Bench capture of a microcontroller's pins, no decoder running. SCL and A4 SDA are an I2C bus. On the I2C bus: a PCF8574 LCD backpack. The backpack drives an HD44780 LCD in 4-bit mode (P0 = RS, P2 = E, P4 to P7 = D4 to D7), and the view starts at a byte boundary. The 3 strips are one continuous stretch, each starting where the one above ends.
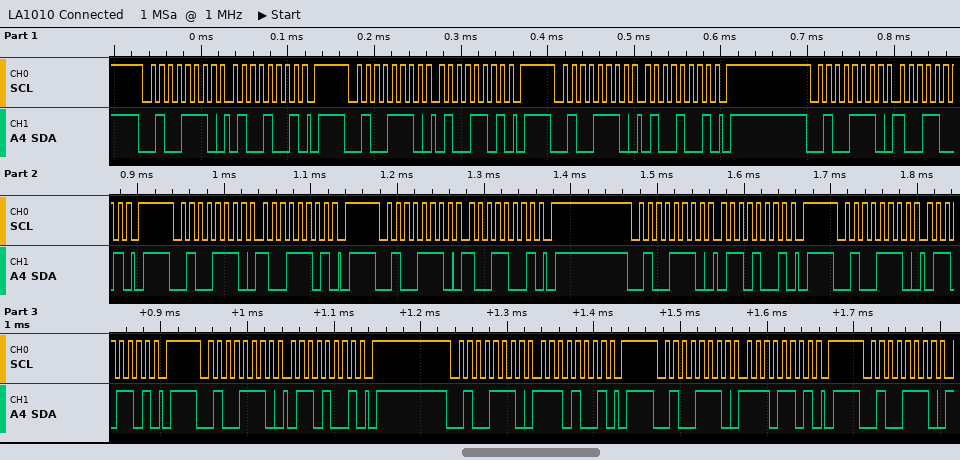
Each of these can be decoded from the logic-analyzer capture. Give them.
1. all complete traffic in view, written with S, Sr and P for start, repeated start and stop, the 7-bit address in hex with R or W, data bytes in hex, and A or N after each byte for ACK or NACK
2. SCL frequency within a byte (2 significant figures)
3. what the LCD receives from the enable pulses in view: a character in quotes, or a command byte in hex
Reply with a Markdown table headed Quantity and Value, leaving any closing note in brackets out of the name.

| Quantity | Value |
|---|---|
| all complete traffic in view, written with S, Sr and P for start, repeated start and stop, the 7-bit address in hex with R or W, data bytes in hex, and A or N after each byte for ACK or NACK | S 27W A 49 A P S 27W A 4D A P S 27W A 49 A P S 27W A 99 A P S 27W A 9D A P S 27W A 99 A P S 27W A 69 A P S 27W A 6D A P S 27W A 69 A P S 27W A E9 A P S 27W A ED A P S 27W A |
| SCL frequency within a byte | 100 kHz |
| what the LCD receives from the enable pulses in view: a character in quotes, or a command byte in hex | 'I' |
